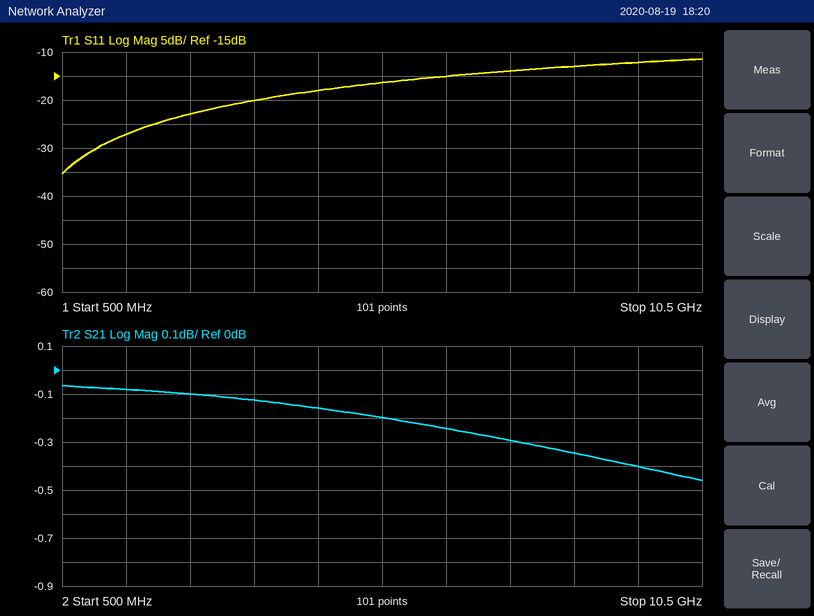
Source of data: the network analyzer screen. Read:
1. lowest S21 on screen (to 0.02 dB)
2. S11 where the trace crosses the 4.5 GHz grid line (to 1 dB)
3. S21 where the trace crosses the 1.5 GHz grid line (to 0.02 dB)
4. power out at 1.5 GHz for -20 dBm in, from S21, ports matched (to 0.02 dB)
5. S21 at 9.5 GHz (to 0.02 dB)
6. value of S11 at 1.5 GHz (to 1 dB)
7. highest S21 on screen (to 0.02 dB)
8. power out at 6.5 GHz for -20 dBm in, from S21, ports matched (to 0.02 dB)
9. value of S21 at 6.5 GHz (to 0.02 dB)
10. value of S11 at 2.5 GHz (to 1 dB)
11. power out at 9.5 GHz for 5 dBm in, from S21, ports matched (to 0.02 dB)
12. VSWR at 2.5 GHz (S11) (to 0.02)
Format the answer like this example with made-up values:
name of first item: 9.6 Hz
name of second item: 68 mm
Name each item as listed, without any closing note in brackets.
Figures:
lowest S21 on screen: -0.46 dB
S11 where the trace crosses the 4.5 GHz grid line: -18 dB
S21 where the trace crosses the 1.5 GHz grid line: -0.08 dB
power out at 1.5 GHz for -20 dBm in, from S21, ports matched: -20.08 dBm
S21 at 9.5 GHz: -0.40 dB
value of S11 at 1.5 GHz: -27 dB
highest S21 on screen: -0.06 dB
power out at 6.5 GHz for -20 dBm in, from S21, ports matched: -20.24 dBm
value of S21 at 6.5 GHz: -0.24 dB
value of S11 at 2.5 GHz: -23 dB
power out at 9.5 GHz for 5 dBm in, from S21, ports matched: 4.60 dBm
VSWR at 2.5 GHz (S11): 1.16
